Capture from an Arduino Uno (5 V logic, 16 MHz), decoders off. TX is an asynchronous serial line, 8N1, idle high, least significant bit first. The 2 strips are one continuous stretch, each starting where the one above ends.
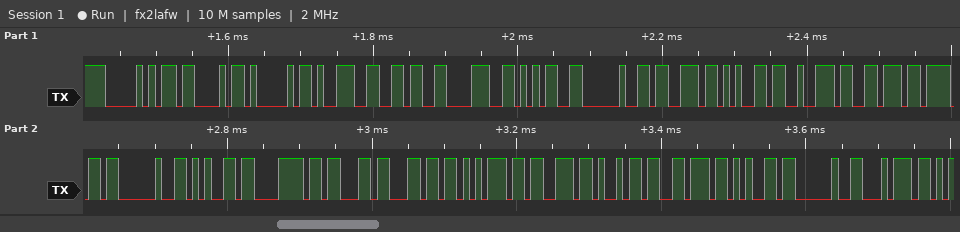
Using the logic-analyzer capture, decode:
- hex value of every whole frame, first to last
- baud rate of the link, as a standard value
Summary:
0x50 0x43 0x41 0x39 0x36 0x38 0x35 0x20 0x73 0x65 0x72 0x76 0x6F 0x20 0x65 0x78 0x63 0x6C 0x75 0x73 0x69 0x76 0x65 0x20 0x74
115200 baud
